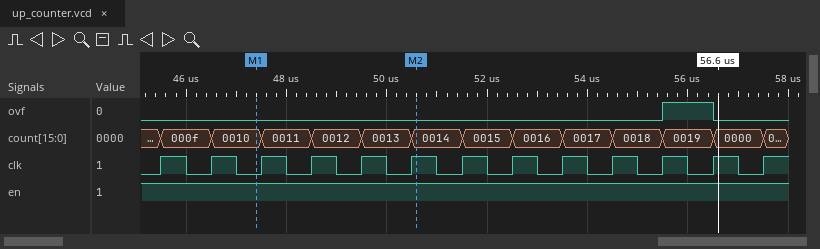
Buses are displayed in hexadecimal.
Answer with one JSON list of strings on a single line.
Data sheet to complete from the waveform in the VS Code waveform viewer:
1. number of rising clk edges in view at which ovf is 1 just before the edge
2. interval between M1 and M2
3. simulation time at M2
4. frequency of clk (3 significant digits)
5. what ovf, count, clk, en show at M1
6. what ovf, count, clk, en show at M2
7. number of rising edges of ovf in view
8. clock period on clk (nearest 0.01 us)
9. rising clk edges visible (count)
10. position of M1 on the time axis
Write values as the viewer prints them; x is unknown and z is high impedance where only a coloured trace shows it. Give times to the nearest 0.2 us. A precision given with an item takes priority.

["1", "3.2 us", "50.6 us", "1.00 MHz", "ovf=0, count=0010, clk=0, en=1", "ovf=0, count=0014, clk=1, en=1", "1", "1 us", "13", "47.4 us"]
